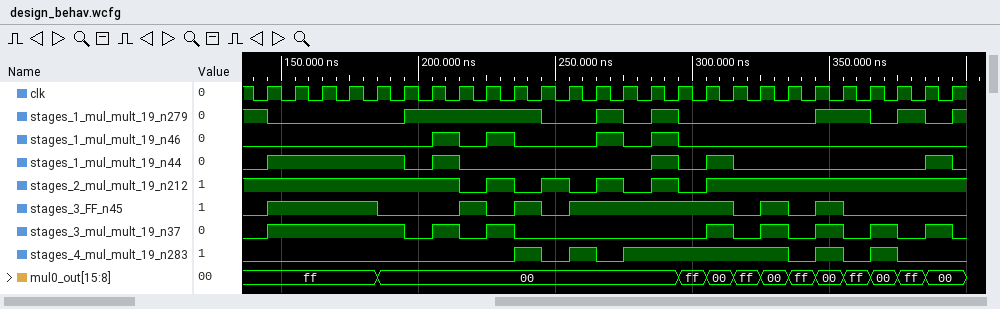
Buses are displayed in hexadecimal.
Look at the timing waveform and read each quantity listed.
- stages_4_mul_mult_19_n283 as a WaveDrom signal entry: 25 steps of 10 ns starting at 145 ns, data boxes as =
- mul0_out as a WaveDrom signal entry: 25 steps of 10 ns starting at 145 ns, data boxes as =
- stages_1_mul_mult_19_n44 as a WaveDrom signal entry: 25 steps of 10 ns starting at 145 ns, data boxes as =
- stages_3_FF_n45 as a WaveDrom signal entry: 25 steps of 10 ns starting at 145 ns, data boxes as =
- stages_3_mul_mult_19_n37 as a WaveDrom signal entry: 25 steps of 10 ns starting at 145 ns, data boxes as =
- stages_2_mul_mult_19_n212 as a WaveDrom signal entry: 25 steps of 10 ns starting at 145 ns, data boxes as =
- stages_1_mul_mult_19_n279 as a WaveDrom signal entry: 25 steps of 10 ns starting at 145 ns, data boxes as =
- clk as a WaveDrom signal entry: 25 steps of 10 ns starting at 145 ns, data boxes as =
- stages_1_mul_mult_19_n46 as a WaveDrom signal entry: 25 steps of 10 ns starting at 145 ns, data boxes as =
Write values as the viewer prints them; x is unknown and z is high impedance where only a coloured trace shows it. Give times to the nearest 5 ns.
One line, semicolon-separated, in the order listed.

{name: 'stages_4_mul_mult_19_n283', wave: '0........10101.....01010.'}; {name: 'mul0_out', wave: '=...=..........==========', data: 'ff 00 ff 00 ff 00 ff 00 ff 00 ff 00'}; {name: 'stages_1_mul_mult_19_n44', wave: '1....010......1010......1'}; {name: 'stages_3_FF_n45', wave: '1...0..10101.....01010...'}; {name: 'stages_3_mul_mult_19_n37', wave: '1....01010......101010101'}; {name: 'stages_2_mul_mult_19_n212', wave: '1......0101010101........'}; {name: 'stages_1_mul_mult_19_n279', wave: '0....1....0.1010....1.010'}; {name: 'clk', wave: 'p........................'}; {name: 'stages_1_mul_mult_19_n46', wave: '0.....1010..1010.........'}
